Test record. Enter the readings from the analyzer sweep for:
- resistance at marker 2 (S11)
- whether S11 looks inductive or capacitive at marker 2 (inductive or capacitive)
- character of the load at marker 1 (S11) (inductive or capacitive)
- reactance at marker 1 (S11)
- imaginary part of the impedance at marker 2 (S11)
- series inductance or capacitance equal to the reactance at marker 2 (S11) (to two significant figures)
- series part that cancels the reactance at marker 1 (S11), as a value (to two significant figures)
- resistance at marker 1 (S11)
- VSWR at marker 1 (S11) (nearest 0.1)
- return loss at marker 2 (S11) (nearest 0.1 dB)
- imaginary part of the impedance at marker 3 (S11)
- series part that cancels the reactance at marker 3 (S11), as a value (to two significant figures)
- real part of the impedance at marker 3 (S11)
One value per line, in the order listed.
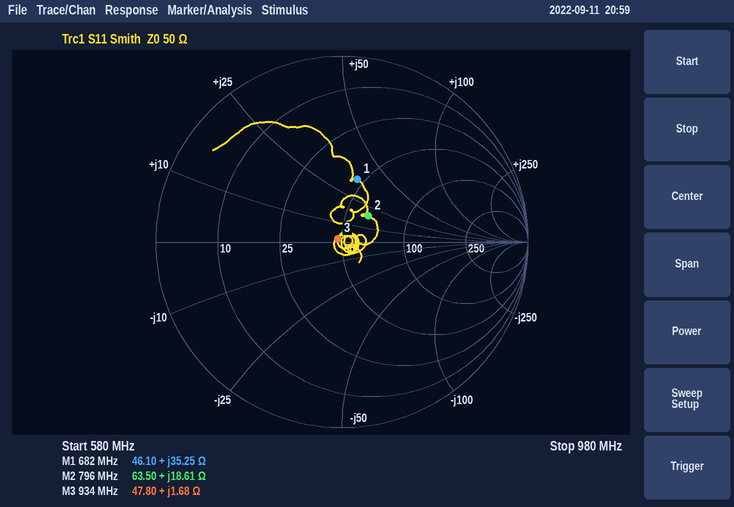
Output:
63.50 Ω
inductive
inductive
+35.25 Ω
+18.61 Ω
3.7 nH
6.6 pF
46.10 Ω
2.1
14.0 dB
+1.68 Ω
100 pF
47.80 Ω
